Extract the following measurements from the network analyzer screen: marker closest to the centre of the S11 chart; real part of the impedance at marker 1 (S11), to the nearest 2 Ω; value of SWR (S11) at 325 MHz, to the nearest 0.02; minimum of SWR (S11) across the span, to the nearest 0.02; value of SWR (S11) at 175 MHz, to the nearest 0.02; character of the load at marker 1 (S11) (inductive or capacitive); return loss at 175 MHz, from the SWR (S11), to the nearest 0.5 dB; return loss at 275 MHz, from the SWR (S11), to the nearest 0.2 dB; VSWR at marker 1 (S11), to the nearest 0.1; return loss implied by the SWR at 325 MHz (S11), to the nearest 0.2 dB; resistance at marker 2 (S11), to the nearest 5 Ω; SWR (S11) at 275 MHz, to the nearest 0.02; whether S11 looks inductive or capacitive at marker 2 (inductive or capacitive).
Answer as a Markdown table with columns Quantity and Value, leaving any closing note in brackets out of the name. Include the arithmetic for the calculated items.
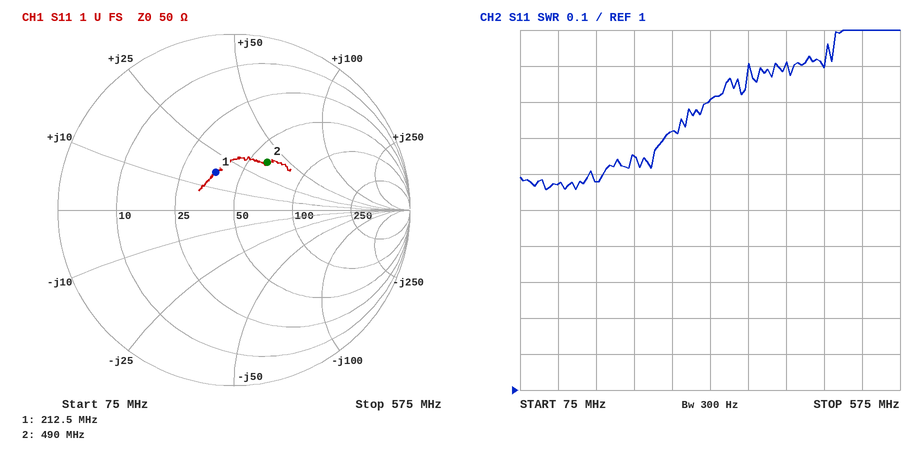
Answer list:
| Quantity | Value |
|---|---|
| marker closest to the centre of the S11 chart | marker 1 |
| real part of the impedance at marker 1 (S11), to the nearest 2 Ω | 38 Ω |
| value of SWR (S11) at 325 MHz, to the nearest 0.02 | 1.80 |
| minimum of SWR (S11) across the span, to the nearest 0.02 | 1.56 |
| value of SWR (S11) at 175 MHz, to the nearest 0.02 | 1.58 |
| character of the load at marker 1 (S11) | inductive |
| return loss at 175 MHz, from the SWR (S11), to the nearest 0.5 dB | −20 log10((1.58 − 1)/(1.58 + 1)) ≈ 13.0 dB |
| return loss at 275 MHz, from the SWR (S11), to the nearest 0.2 dB | −20 log10((1.72 − 1)/(1.72 + 1)) ≈ 11.5 dB, so 11.6 dB to the nearest 0.2 dB |
| VSWR at marker 1 (S11), to the nearest 0.1 | 1.6 |
| return loss implied by the SWR at 325 MHz (S11), to the nearest 0.2 dB | −20 log10((1.8 − 1)/(1.8 + 1)) ≈ 10.9 dB, so 10.8 dB to the nearest 0.2 dB |
| resistance at marker 2 (S11), to the nearest 5 Ω | 60 Ω |
| SWR (S11) at 275 MHz, to the nearest 0.02 | 1.72 |
| whether S11 looks inductive or capacitive at marker 2 | inductive |
